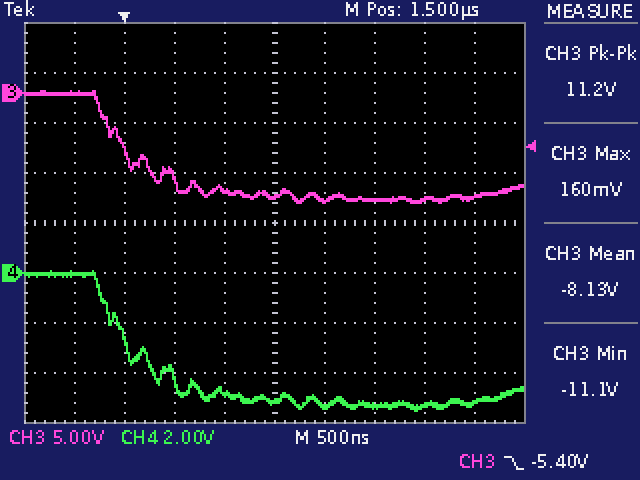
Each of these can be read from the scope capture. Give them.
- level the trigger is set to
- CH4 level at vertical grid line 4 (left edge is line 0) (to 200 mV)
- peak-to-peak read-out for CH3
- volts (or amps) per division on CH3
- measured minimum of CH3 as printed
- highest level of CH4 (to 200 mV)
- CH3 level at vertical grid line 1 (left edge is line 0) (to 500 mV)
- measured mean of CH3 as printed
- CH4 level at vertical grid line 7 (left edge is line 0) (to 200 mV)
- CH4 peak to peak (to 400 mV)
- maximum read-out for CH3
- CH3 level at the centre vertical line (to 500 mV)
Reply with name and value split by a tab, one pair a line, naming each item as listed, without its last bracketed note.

level the trigger is set to	-5.40 V
CH4 level at vertical grid line 4 (left edge is line 0)	-4.8 V
peak-to-peak read-out for CH3	11.2 V
volts (or amps) per division on CH3	5 V
measured minimum of CH3 as printed	-11.1 V
highest level of CH4	0.0 V
CH3 level at vertical grid line 1 (left edge is line 0)	0.0 V
measured mean of CH3 as printed	-8.13 V
CH4 level at vertical grid line 7 (left edge is line 0)	-5.4 V
CH4 peak to peak	5.6 V
maximum read-out for CH3	160 mV
CH3 level at the centre vertical line	-10.5 V
